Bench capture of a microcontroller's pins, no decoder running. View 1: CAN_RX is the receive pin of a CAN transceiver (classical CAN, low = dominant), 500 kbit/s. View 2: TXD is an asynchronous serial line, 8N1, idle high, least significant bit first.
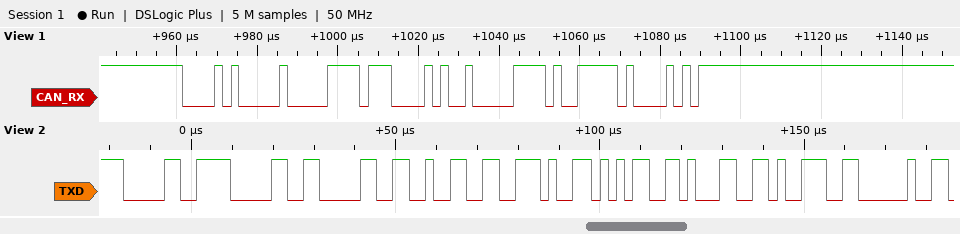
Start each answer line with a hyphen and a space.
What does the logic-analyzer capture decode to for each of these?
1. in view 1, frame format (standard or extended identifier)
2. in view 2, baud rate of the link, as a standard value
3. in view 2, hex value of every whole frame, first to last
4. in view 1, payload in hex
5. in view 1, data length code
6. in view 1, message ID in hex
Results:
- standard
- 500000 baud
- 30 30 30 32 2E 35 31 39 20
- B8 52 0E
- 3
- 0x0A0
